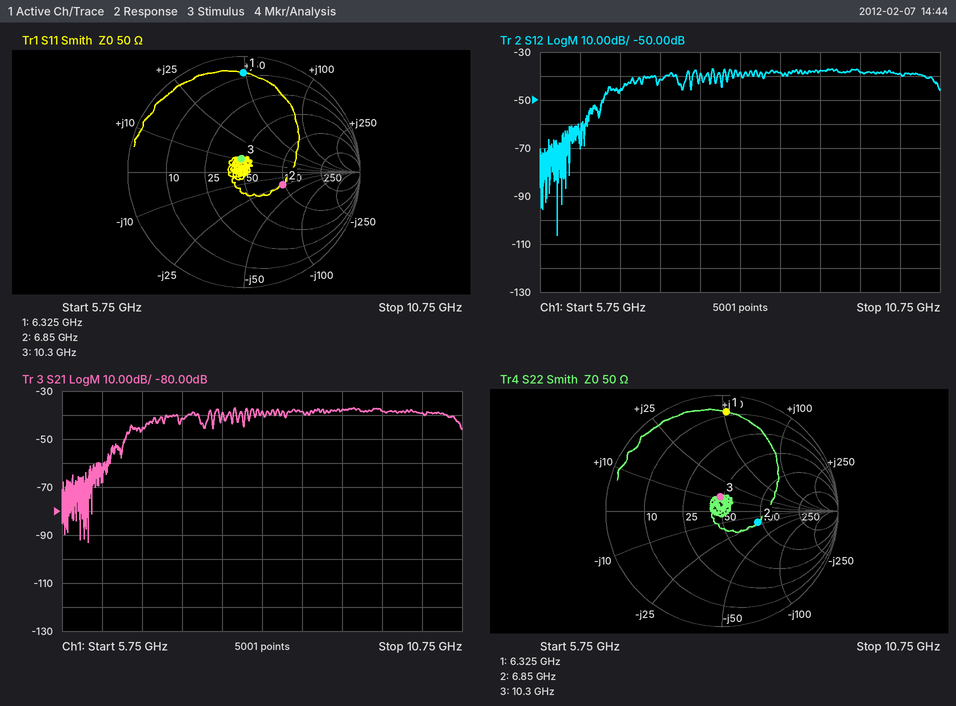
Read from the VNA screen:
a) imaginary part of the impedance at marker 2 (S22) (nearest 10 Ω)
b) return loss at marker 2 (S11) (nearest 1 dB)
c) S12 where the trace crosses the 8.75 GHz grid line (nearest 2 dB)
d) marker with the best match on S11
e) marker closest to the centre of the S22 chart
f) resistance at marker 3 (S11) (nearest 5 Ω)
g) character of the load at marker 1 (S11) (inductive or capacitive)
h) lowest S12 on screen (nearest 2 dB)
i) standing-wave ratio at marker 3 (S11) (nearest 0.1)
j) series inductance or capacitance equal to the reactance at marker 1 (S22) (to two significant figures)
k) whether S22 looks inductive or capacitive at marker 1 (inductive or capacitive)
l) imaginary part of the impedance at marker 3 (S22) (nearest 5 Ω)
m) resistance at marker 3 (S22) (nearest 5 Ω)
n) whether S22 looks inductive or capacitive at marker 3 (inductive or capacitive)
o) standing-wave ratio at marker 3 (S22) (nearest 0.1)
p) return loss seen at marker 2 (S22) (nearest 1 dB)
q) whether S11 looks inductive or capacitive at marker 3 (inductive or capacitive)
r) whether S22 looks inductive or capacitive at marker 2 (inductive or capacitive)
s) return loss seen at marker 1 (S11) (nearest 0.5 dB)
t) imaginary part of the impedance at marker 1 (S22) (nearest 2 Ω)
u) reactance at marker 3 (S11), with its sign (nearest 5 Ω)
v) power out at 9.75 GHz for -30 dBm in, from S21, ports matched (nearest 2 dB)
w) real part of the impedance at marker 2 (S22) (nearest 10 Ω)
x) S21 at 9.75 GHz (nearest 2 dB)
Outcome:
-20 Ω
9 dB
-38 dB
marker 3
marker 3
45 Ω
inductive
-106 dB
1.3
1.3 nH
inductive
+10 Ω
45 Ω
inductive
1.3
10 dB
inductive
capacitive
1.5 dB
+52 Ω
+10 Ω
-68 dBm
90 Ω
-38 dB
